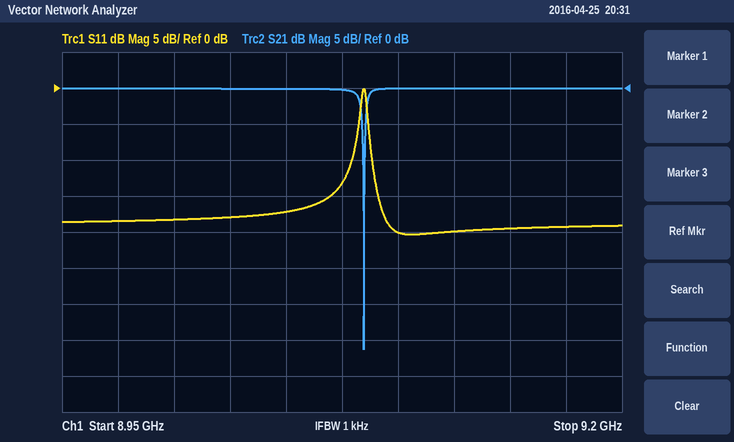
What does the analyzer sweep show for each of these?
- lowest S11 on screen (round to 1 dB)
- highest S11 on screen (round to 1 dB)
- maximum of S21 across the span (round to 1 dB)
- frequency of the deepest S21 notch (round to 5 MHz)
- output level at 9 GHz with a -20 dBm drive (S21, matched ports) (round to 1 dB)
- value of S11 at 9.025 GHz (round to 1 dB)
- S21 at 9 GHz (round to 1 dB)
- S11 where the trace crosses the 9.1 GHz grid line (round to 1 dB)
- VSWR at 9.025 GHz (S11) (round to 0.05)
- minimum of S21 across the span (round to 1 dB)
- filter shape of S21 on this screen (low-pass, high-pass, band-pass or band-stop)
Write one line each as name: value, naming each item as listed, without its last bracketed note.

lowest S11 on screen: -20 dB
highest S11 on screen: 0 dB
maximum of S21 across the span: 0 dB
frequency of the deepest S21 notch: 9.085 GHz
output level at 9 GHz with a -20 dBm drive (S21, matched ports): -20 dBm
value of S11 at 9.025 GHz: -18 dB
S21 at 9 GHz: 0 dB
S11 where the trace crosses the 9.1 GHz grid line: -20 dB
VSWR at 9.025 GHz (S11): 1.30
minimum of S21 across the span: -36 dB
filter shape of S21 on this screen: band-stop
